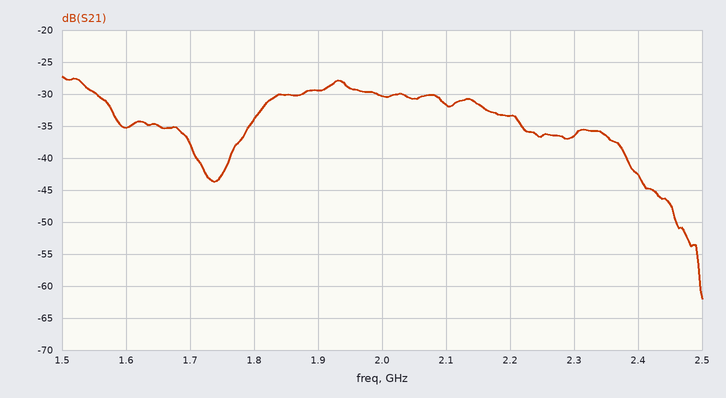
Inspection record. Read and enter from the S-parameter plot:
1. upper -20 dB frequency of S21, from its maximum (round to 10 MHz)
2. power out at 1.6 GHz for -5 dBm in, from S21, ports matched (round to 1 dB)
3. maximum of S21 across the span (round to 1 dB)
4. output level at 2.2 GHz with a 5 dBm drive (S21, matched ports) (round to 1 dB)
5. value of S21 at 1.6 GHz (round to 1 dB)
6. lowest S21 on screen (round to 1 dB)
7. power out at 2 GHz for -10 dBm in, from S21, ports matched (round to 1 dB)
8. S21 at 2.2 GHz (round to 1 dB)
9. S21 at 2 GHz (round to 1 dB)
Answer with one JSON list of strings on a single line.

["2.45 GHz", "-40 dBm", "-27 dB", "-28 dBm", "-35 dB", "-62 dB", "-40 dBm", "-33 dB", "-30 dB"]
